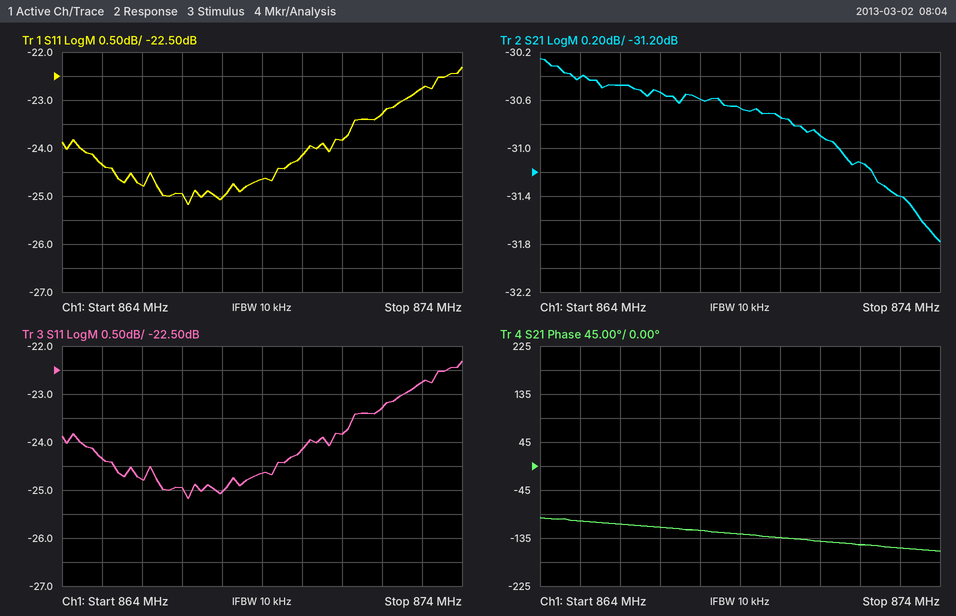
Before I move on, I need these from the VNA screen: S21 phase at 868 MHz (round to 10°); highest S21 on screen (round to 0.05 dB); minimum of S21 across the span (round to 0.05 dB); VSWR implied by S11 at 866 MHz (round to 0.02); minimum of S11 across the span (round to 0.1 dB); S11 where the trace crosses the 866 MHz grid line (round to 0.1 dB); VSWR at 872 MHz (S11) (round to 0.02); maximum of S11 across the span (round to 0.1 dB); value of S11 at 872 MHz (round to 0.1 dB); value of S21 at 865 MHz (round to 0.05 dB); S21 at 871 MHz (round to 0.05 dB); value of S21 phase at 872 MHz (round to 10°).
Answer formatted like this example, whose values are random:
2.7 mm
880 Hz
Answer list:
-120°
-30.25 dB
-31.80 dB
1.12
-25.2 dB
-24.8 dB
1.14
-22.3 dB
-23.3 dB
-30.40 dB
-30.90 dB
-150°
